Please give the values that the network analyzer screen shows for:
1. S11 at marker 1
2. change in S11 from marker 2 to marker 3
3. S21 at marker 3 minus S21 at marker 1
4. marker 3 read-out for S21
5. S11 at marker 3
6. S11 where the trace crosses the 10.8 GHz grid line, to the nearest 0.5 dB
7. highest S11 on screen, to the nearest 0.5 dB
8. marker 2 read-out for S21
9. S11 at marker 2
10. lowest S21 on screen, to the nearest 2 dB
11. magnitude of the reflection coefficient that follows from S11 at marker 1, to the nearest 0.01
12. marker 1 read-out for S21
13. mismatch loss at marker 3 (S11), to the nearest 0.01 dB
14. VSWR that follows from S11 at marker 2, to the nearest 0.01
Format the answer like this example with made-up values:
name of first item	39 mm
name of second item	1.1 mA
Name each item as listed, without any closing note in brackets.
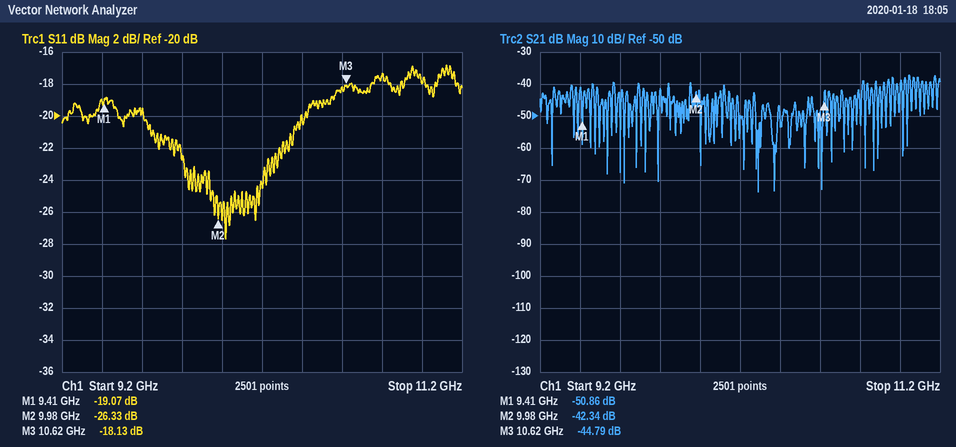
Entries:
S11 at marker 1	-19.07 dB
change in S11 from marker 2 to marker 3	8.20 dB
S21 at marker 3 minus S21 at marker 1	6.07 dB
marker 3 read-out for S21	-44.79 dB
S11 at marker 3	-18.13 dB
S11 where the trace crosses the 10.8 GHz grid line, to the nearest 0.5 dB	-17.5 dB
highest S11 on screen, to the nearest 0.5 dB	-17.0 dB
marker 2 read-out for S21	-42.34 dB
S11 at marker 2	-26.33 dB
lowest S21 on screen, to the nearest 2 dB	-74 dB
magnitude of the reflection coefficient that follows from S11 at marker 1, to the nearest 0.01	0.11
marker 1 read-out for S21	-50.86 dB
mismatch loss at marker 3 (S11), to the nearest 0.01 dB	0.07 dB
VSWR that follows from S11 at marker 2, to the nearest 0.01	1.10
